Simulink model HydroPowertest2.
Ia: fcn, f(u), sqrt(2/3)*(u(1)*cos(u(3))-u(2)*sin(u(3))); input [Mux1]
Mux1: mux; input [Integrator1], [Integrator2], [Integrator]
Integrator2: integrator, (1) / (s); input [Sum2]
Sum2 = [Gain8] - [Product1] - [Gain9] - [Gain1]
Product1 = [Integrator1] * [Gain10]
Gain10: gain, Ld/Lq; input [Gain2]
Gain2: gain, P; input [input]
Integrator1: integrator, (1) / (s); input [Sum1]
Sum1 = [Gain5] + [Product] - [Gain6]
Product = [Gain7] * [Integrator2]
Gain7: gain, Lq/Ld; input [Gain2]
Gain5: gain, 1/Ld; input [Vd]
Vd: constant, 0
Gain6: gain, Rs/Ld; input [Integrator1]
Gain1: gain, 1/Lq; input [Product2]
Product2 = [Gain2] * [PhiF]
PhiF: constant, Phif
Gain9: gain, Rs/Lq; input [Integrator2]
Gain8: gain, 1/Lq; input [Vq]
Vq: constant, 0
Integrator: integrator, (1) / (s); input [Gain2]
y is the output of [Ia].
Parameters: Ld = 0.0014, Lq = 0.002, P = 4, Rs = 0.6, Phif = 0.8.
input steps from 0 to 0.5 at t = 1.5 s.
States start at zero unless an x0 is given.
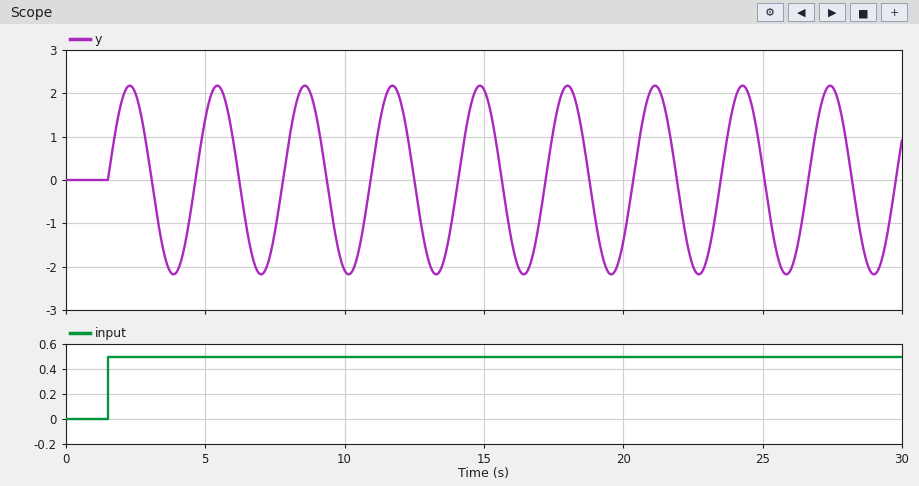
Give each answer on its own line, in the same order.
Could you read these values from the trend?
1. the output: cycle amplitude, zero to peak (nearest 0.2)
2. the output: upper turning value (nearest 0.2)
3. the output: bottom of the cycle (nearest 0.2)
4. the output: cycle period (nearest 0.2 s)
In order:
2.2
2.2
-2.2
3.2 s
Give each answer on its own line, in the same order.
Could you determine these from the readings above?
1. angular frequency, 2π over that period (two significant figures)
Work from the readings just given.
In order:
2.0 rad/s
